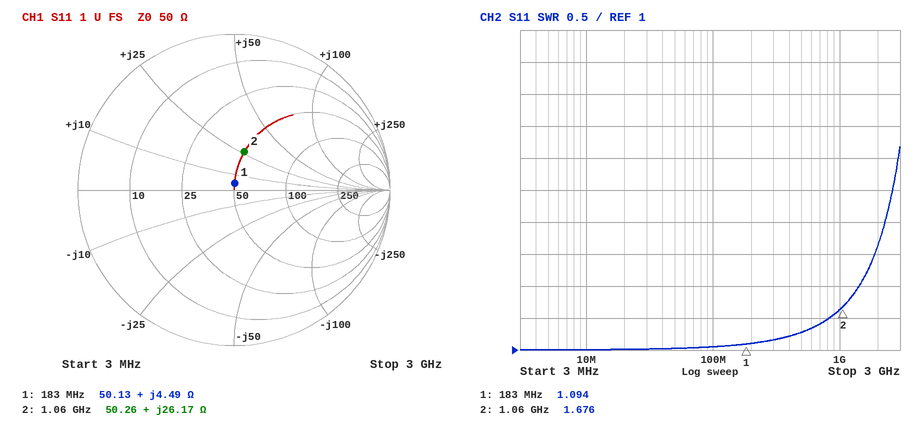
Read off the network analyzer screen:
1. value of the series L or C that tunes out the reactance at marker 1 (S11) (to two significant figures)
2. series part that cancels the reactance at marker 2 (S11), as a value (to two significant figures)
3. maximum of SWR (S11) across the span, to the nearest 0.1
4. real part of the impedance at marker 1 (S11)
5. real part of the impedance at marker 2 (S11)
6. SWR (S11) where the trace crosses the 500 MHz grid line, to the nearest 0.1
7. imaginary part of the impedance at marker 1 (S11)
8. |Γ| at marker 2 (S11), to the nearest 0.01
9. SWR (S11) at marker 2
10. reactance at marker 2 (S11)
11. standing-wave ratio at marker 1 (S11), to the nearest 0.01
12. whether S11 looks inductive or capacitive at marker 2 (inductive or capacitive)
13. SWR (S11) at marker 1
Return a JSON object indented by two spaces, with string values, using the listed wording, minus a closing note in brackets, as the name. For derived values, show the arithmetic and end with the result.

{
  "value of the series L or C that tunes out the reactance at marker 1 (S11)": "C = 1/(2π × 183 MHz × 4.49 Ω) ≈ 194 pF, so 190 pF to two significant figures",
  "series part that cancels the reactance at marker 2 (S11), as a value": "C = 1/(2π × 1.06 GHz × 26.17 Ω) ≈ 5.7 pF",
  "maximum of SWR (S11) across the span, to the nearest 0.1": "4.2",
  "real part of the impedance at marker 1": "50.13 Ω",
  "real part of the impedance at marker 2": "50.26 Ω",
  "SWR (S11) where the trace crosses the 500 MHz grid line, to the nearest 0.1": "1.3",
  "imaginary part of the impedance at marker 1": "+4.49 Ω",
  "|Γ| at marker 2 (S11), to the nearest 0.01": "0.25",
  "SWR (S11) at marker 2": "1.676",
  "reactance at marker 2": "+26.17 Ω",
  "standing-wave ratio at marker 1 (S11), to the nearest 0.01": "1.09",
  "whether S11 looks inductive or capacitive at marker 2": "inductive",
  "SWR (S11) at marker 1": "1.094"
}
